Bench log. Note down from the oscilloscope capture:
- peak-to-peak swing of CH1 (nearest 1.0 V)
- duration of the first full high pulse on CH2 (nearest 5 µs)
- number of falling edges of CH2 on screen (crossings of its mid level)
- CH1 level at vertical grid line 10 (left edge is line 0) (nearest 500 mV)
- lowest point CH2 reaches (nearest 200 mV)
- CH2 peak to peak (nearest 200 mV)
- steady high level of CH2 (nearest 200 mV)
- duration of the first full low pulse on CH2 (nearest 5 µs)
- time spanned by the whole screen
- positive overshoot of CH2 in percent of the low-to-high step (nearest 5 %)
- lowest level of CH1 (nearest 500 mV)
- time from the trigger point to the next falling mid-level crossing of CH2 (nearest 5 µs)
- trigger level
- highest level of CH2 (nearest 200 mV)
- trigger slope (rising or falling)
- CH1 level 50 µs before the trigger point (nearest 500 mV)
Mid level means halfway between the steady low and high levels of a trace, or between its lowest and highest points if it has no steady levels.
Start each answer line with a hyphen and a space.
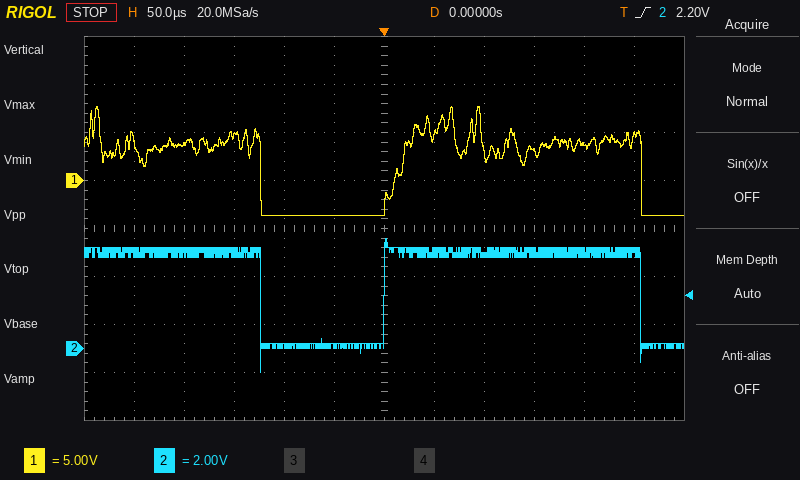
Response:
- 11.0 V
- 255 µs
- 2
- 3.5 V
- -1.0 V
- 5.6 V
- 4.0 V
- 125 µs
- 600 µs
- 15 %
- -3.5 V
- 255 µs
- 2.20 V
- 4.6 V
- rising
- -3.5 V
